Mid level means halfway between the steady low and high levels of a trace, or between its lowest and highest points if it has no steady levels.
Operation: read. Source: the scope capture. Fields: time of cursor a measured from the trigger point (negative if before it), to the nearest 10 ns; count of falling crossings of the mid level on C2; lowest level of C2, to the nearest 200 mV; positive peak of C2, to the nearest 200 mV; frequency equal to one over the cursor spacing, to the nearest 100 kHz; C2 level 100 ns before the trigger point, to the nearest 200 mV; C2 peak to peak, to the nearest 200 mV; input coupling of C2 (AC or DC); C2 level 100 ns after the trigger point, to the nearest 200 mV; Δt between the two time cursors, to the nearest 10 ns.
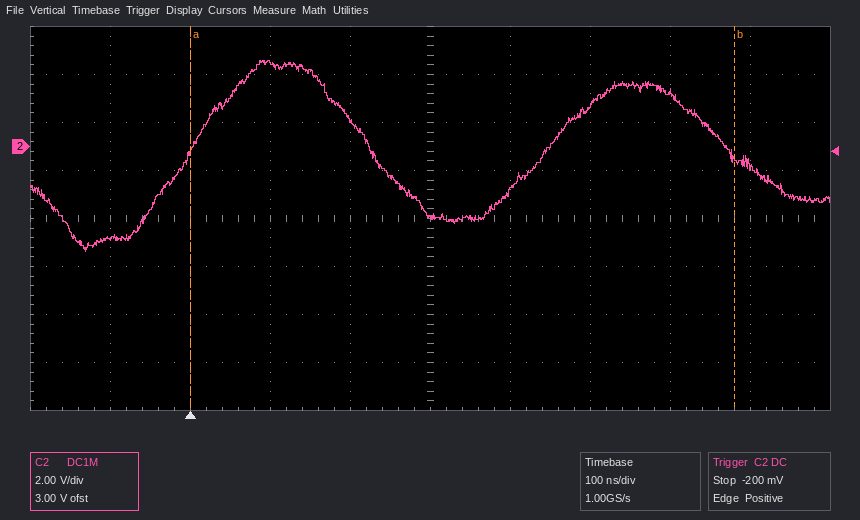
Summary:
0 ns
2
-4.4 V
3.6 V
1.5 MHz
-3.8 V
8.0 V
DC
3.4 V
680 ns
